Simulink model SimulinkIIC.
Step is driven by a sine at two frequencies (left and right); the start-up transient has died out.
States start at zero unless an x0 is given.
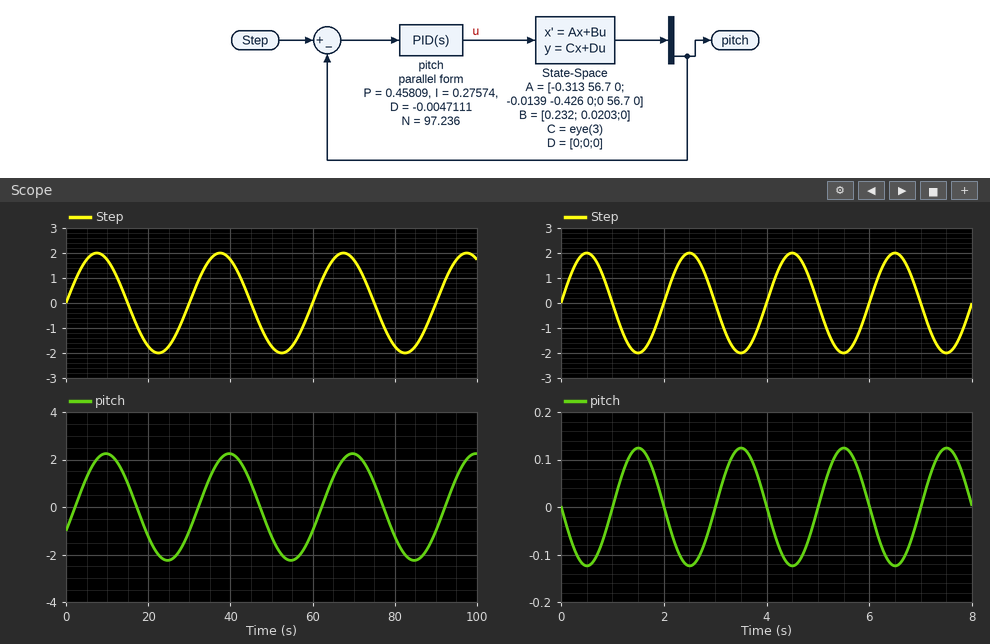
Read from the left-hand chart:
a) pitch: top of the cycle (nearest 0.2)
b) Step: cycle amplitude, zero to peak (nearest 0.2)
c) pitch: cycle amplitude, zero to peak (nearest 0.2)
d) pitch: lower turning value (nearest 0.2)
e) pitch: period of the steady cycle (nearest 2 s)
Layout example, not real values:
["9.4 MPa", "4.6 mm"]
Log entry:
["2.2", "2.0", "2.2", "-2.2", "30 s"]
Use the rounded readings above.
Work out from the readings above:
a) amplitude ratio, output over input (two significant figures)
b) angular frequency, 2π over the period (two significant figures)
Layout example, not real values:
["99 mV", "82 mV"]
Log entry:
["1.1", "0.21 rad/s"]
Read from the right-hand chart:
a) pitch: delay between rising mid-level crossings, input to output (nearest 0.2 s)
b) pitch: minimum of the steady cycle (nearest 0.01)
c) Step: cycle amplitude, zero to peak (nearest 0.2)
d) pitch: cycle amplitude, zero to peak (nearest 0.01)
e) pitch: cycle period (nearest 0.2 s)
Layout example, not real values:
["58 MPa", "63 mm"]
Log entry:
["1.0 s", "-0.12", "2.0", "0.12", "2.0 s"]
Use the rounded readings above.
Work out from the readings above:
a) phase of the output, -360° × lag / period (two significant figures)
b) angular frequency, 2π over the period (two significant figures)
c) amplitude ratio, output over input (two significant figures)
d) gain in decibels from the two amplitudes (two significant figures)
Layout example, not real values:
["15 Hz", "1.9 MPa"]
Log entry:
["-180°", "3.1 rad/s", "0.060", "-24 dB"]
